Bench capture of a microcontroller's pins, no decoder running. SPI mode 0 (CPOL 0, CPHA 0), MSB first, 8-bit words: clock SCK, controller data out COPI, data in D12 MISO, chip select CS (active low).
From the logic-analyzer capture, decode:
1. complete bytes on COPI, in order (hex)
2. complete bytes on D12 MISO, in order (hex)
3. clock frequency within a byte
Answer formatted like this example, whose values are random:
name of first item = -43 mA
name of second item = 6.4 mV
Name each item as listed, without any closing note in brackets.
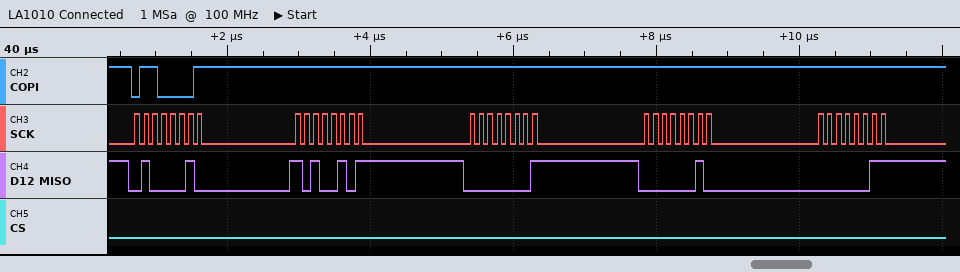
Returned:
complete bytes on COPI, in order = 61 FF FF FF FF
complete bytes on D12 MISO, in order = 42 A5 01 02 03
clock frequency within a byte = 8 MHz
